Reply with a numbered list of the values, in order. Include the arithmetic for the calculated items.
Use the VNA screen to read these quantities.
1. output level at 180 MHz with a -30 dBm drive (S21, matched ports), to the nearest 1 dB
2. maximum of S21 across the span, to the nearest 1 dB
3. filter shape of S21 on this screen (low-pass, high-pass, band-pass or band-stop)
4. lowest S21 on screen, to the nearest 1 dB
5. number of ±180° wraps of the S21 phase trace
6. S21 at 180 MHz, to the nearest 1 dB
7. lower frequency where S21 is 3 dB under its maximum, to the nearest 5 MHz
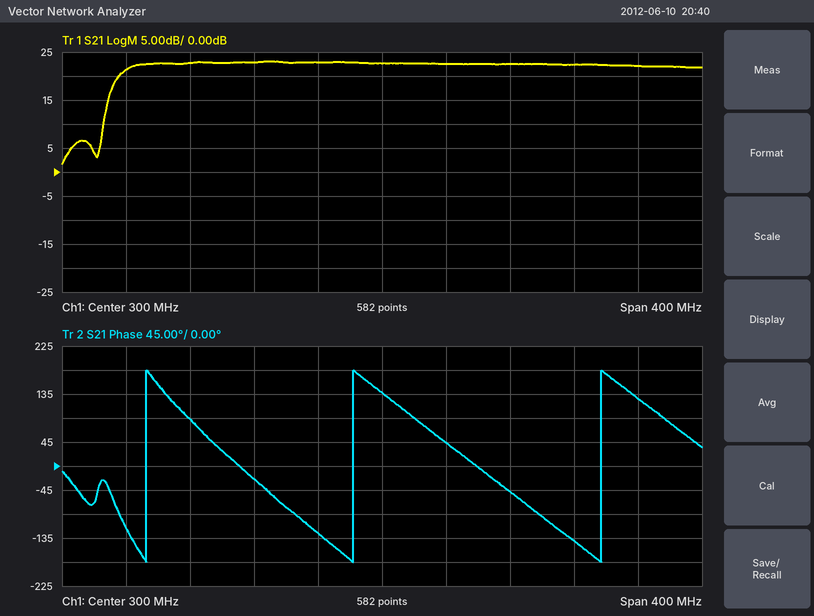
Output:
1. -30 dBm + (23 dB) = -7 dBm
2. 23 dB
3. high-pass
4. 2 dB
5. 3
6. 23 dB
7. 135 MHz
